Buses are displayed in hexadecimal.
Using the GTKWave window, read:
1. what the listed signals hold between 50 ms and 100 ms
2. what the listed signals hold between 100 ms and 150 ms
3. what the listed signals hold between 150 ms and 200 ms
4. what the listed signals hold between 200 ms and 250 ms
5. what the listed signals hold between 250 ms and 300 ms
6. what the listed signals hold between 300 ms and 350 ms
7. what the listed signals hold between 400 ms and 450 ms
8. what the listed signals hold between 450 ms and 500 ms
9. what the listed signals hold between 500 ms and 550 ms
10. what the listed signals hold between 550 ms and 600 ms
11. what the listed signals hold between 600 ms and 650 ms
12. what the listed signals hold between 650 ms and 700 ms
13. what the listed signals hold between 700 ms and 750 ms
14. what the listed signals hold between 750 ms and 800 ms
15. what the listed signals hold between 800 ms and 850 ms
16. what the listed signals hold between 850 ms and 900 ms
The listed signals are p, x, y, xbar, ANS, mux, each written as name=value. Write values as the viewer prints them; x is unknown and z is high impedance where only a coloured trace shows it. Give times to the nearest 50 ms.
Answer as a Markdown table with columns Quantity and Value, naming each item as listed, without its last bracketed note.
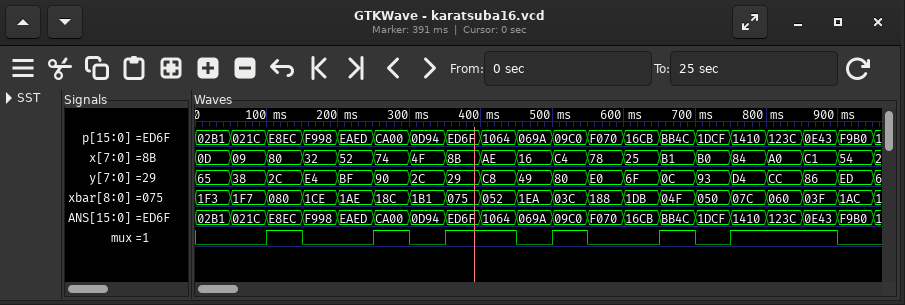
| Quantity | Value |
|---|---|
| what the listed signals hold between 50 ms and 100 ms | p=021C, x=09, y=38, xbar=1F7, ANS=021C, mux=0 |
| what the listed signals hold between 100 ms and 150 ms | p=E8EC, x=80, y=2C, xbar=080, ANS=E8EC, mux=1 |
| what the listed signals hold between 150 ms and 200 ms | p=F998, x=32, y=E4, xbar=1CE, ANS=F998, mux=0 |
| what the listed signals hold between 200 ms and 250 ms | p=EAED, x=52, y=BF, xbar=1AE, ANS=EAED, mux=0 |
| what the listed signals hold between 250 ms and 300 ms | p=CA00, x=74, y=90, xbar=18C, ANS=CA00, mux=1 |
| what the listed signals hold between 300 ms and 350 ms | p=0D94, x=4F, y=2C, xbar=1B1, ANS=0D94, mux=0 |
| what the listed signals hold between 400 ms and 450 ms | p=1064, x=AE, y=C8, xbar=052, ANS=1064, mux=1 |
| what the listed signals hold between 450 ms and 500 ms | p=069A, x=16, y=49, xbar=1EA, ANS=069A, mux=0 |
| what the listed signals hold between 500 ms and 550 ms | p=09C0, x=C4, y=80, xbar=03C, ANS=09C0, mux=1 |
| what the listed signals hold between 550 ms and 600 ms | p=F070, x=78, y=E0, xbar=188, ANS=F070, mux=0 |
| what the listed signals hold between 600 ms and 650 ms | p=16CB, x=25, y=6F, xbar=1DB, ANS=16CB, mux=0 |
| what the listed signals hold between 650 ms and 700 ms | p=BB4C, x=B1, y=0C, xbar=04F, ANS=BB4C, mux=1 |
| what the listed signals hold between 700 ms and 750 ms | p=1DCF, x=B0, y=93, xbar=050, ANS=1DCF, mux=0 |
| what the listed signals hold between 750 ms and 800 ms | p=1410, x=84, y=D4, xbar=07C, ANS=1410, mux=1 |
| what the listed signals hold between 800 ms and 850 ms | p=123C, x=A0, y=CC, xbar=060, ANS=123C, mux=1 |
| what the listed signals hold between 850 ms and 900 ms | p=0E43, x=C1, y=86, xbar=03F, ANS=0E43, mux=1 |
